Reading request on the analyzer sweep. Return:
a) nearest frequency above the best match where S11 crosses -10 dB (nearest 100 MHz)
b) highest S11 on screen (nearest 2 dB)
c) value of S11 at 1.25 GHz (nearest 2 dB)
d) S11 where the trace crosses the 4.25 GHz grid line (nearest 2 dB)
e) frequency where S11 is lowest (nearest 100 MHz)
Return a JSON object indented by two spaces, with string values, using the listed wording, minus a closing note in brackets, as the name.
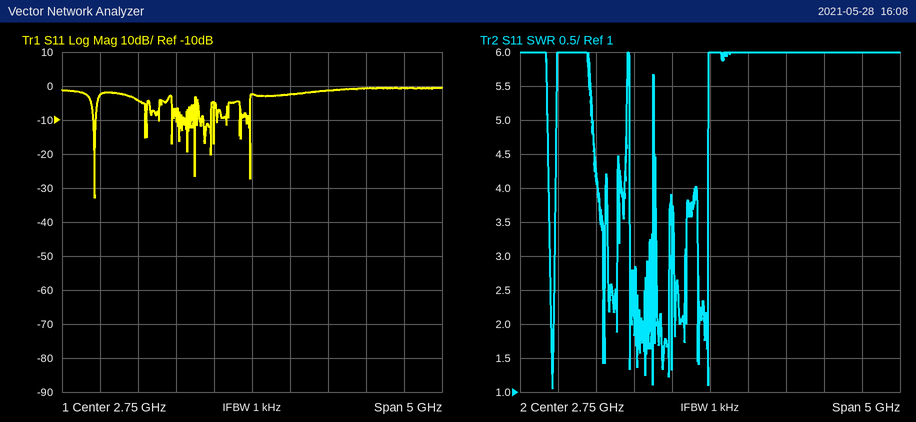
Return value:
{
  "nearest frequency above the best match where S11 crosses -10 dB": "700 MHz",
  "highest S11 on screen": "0 dB",
  "value of S11 at 1.25 GHz": "-4 dB",
  "S11 where the trace crosses the 4.25 GHz grid line": "0 dB",
  "frequency where S11 is lowest": "700 MHz"
}
